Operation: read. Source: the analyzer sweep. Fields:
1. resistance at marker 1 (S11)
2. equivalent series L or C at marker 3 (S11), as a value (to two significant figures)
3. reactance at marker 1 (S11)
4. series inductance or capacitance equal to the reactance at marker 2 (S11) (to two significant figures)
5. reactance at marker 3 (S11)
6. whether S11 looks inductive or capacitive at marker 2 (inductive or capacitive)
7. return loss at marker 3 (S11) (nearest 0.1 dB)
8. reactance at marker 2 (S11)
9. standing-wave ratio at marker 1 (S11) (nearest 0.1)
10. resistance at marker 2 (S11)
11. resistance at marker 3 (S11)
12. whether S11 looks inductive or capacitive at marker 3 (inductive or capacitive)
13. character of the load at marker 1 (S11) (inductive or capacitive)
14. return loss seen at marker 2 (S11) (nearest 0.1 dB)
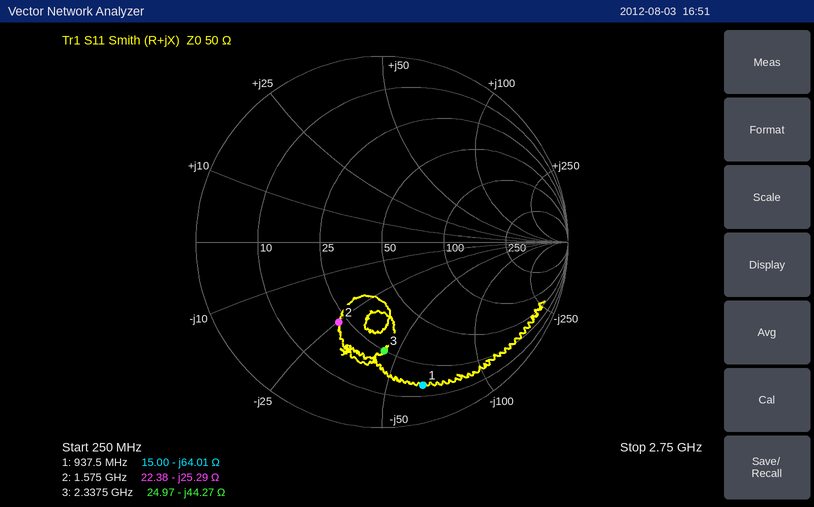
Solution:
15.00 Ω
1.5 pF
-64.01 Ω
4.0 pF
-44.27 Ω
capacitive
4.7 dB
-25.29 Ω
9.0
22.38 Ω
24.97 Ω
capacitive
capacitive
6.2 dB
